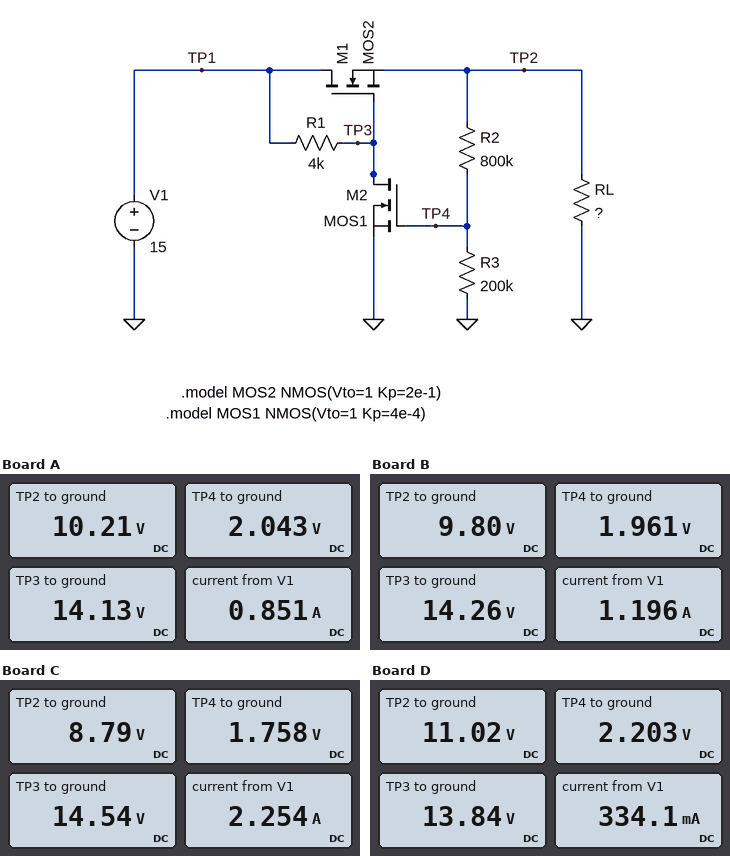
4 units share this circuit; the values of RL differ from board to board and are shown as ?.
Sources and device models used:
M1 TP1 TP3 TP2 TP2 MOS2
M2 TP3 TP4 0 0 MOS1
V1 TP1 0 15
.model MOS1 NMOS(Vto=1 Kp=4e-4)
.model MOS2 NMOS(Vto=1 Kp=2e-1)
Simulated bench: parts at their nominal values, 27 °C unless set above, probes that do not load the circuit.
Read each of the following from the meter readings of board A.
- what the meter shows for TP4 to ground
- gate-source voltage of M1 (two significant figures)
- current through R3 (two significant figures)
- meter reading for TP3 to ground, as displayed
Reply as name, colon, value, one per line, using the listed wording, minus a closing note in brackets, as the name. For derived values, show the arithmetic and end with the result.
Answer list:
what the meter shows for TP4 to ground: 2.043 V
gate-source voltage of M1: 14.13 V - 10.21 V = 3.9 V
current through R3: (2.043 V) / 200 kΩ = 10 µA
meter reading for TP3 to ground, as displayed: 14.13 V
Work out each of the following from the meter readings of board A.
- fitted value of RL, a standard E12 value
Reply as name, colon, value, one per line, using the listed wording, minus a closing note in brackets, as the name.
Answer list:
fitted value of RL, a standard E12 value: 12 Ω
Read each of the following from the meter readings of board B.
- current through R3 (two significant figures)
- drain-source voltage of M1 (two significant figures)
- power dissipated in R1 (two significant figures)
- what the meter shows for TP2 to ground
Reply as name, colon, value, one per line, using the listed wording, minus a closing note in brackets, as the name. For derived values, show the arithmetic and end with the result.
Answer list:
current through R3: (1.961 V) / 200 kΩ = 9.8 µA
drain-source voltage of M1: 15 V - 9.8 V = 5.2 V
power dissipated in R1: (15 V - 14.26 V)^2 / 4 kΩ = 140 µW
what the meter shows for TP2 to ground: 9.80 V
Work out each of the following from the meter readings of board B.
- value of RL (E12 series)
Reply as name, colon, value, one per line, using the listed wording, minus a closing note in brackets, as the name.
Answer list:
value of RL: 8.2 Ω
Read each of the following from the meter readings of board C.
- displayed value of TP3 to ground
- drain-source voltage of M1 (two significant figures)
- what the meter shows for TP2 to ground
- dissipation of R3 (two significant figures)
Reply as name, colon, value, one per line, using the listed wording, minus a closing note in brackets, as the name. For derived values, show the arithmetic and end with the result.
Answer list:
displayed value of TP3 to ground: 14.54 V
drain-source voltage of M1: 15 V - 8.79 V = 6.2 V
what the meter shows for TP2 to ground: 8.79 V
dissipation of R3: (1.758 V)^2 / 200 kΩ = 15 µW
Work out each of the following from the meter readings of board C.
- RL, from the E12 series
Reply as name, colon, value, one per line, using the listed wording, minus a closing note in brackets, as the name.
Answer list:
RL, from the E12 series: 3.9 Ω
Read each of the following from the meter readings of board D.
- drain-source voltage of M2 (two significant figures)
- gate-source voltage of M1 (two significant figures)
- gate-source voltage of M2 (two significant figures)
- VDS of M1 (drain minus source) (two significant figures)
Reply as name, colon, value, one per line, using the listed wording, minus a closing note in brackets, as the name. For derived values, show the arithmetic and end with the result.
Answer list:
drain-source voltage of M2: 13.84 V = 14 V
gate-source voltage of M1: 13.84 V - 11.02 V = 2.8 V
gate-source voltage of M2: 2.203 V = 2.2 V
VDS of M1 (drain minus source): 15 V - 11.02 V = 4.0 V
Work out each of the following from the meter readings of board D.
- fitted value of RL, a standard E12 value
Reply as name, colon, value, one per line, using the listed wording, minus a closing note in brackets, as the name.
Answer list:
fitted value of RL, a standard E12 value: 33 Ω
